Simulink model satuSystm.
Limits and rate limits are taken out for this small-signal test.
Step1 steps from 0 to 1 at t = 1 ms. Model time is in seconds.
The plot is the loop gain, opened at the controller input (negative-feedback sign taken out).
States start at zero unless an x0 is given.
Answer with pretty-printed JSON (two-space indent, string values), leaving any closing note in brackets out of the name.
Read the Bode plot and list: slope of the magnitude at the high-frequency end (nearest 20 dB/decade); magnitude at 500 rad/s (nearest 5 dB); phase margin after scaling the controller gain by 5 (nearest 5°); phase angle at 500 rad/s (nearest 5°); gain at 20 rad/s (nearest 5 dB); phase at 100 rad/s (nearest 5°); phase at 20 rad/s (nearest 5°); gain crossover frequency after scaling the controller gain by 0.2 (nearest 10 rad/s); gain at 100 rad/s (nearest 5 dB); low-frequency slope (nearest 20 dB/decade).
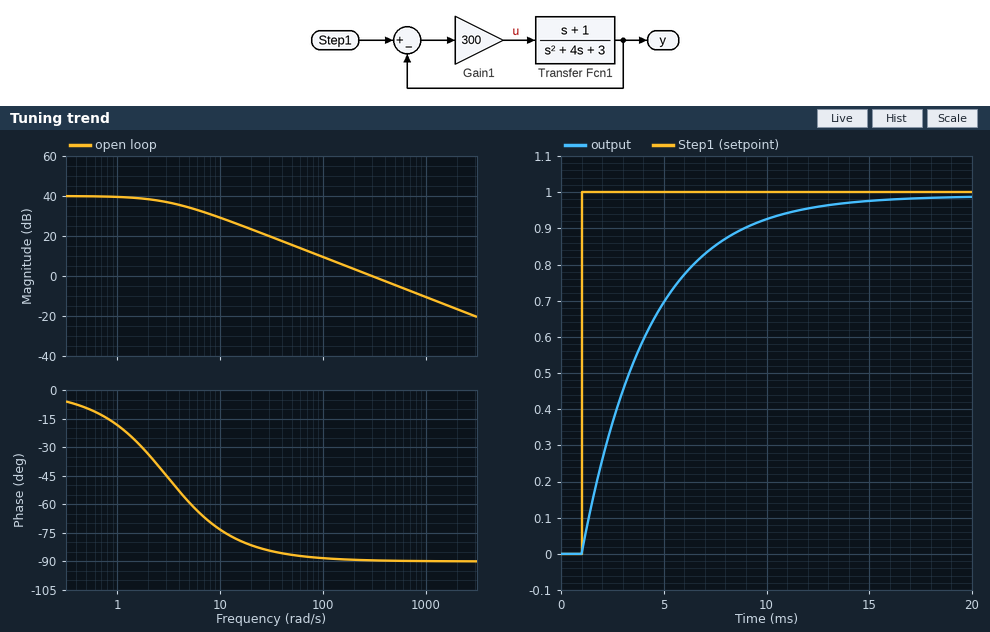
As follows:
{
  "slope of the magnitude at the high-frequency end": "-20 dB/decade",
  "magnitude at 500 rad/s": "-5 dB",
  "phase margin after scaling the controller gain by 5": "90°",
  "phase angle at 500 rad/s": "-90°",
  "gain at 20 rad/s": "25 dB",
  "phase at 100 rad/s": "-90°",
  "phase at 20 rad/s": "-80°",
  "gain crossover frequency after scaling the controller gain by 0.2": "60 rad/s",
  "gain at 100 rad/s": "10 dB",
  "low-frequency slope": "0 dB/decade"
}
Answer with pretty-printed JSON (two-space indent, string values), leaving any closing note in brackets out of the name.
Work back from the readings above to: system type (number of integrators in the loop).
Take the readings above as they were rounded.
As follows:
{
  "system type": "0"
}
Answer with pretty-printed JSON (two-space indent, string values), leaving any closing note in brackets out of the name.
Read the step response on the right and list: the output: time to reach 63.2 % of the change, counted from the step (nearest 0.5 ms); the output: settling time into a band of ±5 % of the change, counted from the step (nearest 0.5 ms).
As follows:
{
  "the output: time to reach 63.2 % of the change, counted from the step": "3.5 ms",
  "the output: settling time into a band of ±5 % of the change, counted from the step": "10.0 ms"
}
